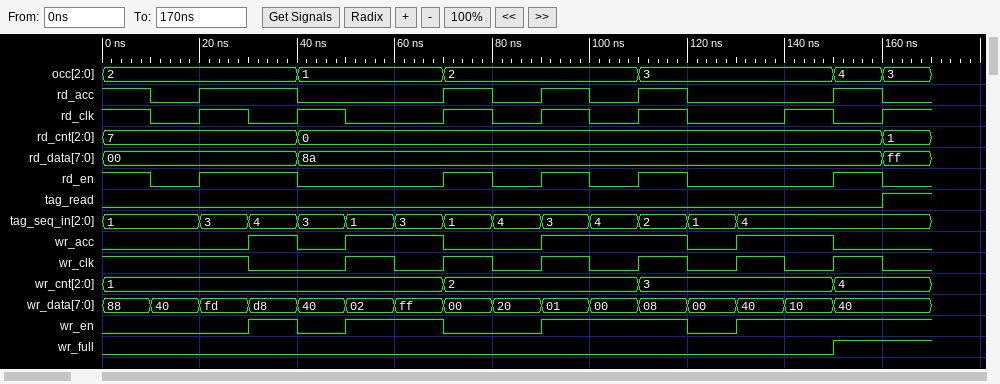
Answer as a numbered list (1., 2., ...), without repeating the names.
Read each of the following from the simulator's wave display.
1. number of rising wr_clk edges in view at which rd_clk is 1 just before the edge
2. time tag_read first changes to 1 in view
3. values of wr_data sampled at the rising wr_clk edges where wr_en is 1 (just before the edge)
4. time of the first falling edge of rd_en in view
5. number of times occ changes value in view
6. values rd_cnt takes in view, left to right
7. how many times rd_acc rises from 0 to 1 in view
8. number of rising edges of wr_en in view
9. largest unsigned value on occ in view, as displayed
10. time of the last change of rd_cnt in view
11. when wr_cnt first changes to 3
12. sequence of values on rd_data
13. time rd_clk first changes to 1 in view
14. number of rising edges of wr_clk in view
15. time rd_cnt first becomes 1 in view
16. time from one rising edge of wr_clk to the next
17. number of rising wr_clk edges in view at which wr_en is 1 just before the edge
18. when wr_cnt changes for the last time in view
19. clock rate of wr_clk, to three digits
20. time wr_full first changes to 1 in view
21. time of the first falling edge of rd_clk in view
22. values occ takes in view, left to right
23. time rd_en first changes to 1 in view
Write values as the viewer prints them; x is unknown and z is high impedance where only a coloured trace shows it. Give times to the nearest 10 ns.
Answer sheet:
1. 2
2. 160 ns
3. ff, 00, 10
4. 10 ns
5. 5
6. 7, 0, 1
7. 5
8. 4
9. 4
10. 160 ns
11. 110 ns
12. 00, 8a, ff
13. 20 ns
14. 6
15. 160 ns
16. 20 ns
17. 3
18. 150 ns
19. 50.0 MHz
20. 150 ns
21. 10 ns
22. 2, 1, 2, 3, 4, 3
23. 20 ns
